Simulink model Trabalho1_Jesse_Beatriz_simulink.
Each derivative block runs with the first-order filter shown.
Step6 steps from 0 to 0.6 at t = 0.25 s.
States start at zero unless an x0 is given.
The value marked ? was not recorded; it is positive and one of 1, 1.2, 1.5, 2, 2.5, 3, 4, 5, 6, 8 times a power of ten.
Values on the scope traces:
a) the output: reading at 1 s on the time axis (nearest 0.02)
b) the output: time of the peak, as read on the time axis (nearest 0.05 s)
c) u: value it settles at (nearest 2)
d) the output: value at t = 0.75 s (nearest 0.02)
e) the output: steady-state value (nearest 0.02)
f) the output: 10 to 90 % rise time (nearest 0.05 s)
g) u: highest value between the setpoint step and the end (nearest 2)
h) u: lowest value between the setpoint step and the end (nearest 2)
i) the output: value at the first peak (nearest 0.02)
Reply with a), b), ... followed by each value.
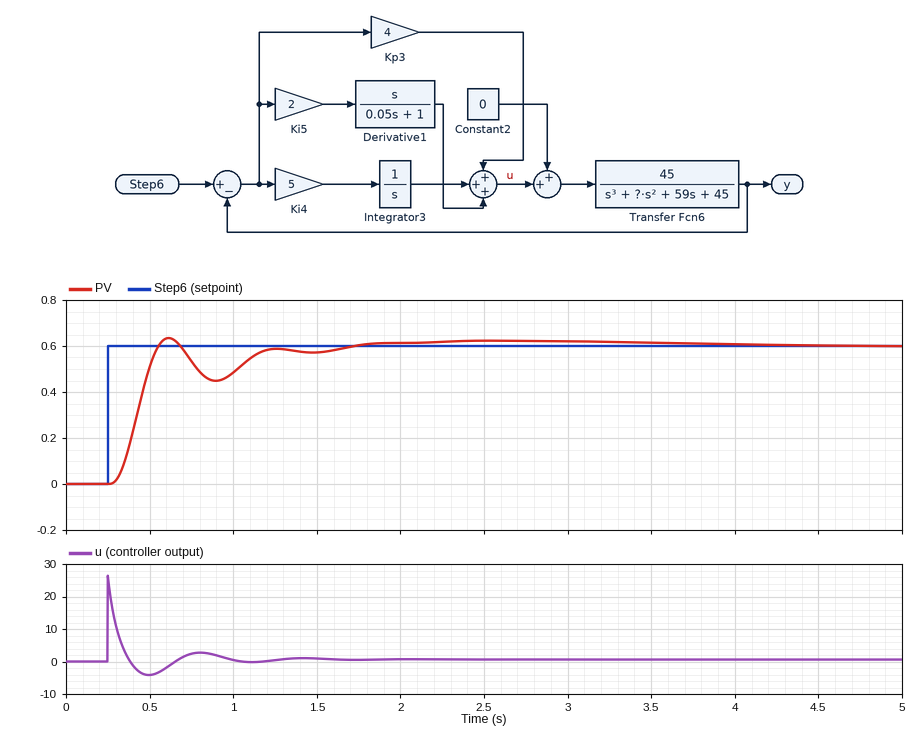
a) 0.48
b) 0.60 s
c) 0
d) 0.54
e) 0.60
f) 0.20 s
g) 26
h) -4
i) 0.64
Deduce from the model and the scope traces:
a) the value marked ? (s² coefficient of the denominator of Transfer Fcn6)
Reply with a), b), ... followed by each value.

a) 12
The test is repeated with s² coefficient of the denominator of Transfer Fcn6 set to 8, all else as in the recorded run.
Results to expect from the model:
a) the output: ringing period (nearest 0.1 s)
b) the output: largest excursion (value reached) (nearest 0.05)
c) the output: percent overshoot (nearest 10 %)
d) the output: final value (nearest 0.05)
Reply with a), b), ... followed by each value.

a) 0.6 s
b) 0.70
c) 20 %
d) 0.60
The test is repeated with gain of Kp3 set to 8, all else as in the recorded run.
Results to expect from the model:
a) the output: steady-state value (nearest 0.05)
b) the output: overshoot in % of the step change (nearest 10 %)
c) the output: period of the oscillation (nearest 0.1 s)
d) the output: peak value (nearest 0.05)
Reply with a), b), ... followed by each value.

a) 0.60
b) 30 %
c) 0.6 s
d) 0.75
